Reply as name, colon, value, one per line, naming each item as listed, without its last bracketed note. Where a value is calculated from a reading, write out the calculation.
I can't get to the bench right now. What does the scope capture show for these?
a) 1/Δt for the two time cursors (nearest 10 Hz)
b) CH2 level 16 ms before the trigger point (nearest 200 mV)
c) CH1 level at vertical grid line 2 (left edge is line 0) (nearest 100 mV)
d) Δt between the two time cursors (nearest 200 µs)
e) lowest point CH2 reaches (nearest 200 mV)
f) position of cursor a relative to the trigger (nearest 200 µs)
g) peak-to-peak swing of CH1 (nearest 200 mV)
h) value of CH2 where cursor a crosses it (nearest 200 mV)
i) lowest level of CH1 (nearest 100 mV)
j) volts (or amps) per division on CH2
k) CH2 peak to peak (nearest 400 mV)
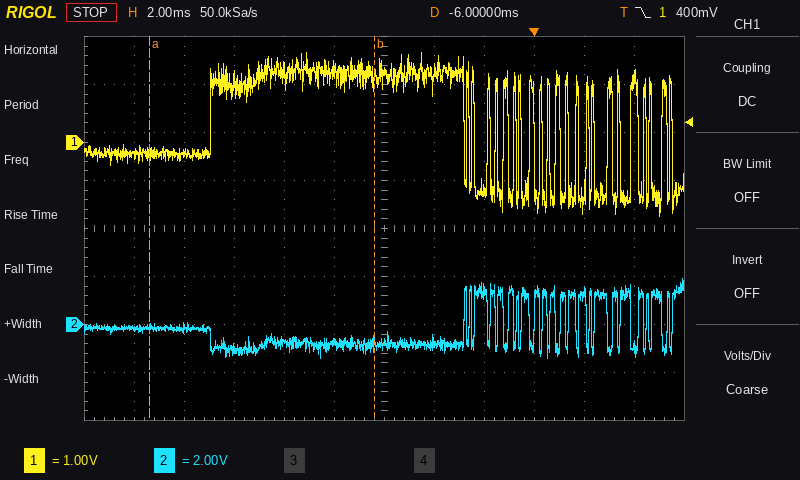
1/Δt for the two time cursors: 1 / 9.0 ms ≈ 110 Hz
CH2 level 16 ms before the trigger point: -200 mV
CH1 level at vertical grid line 2 (left edge is line 0): -200 mV
Δt between the two time cursors: 9.0 ms
lowest point CH2 reaches: -1.4 V
position of cursor a relative to the trigger: -15.4 ms
peak-to-peak swing of CH1: 3.4 V
value of CH2 where cursor a crosses it: 0.0 V
lowest level of CH1: -1.5 V
volts (or amps) per division on CH2: 2 V
CH2 peak to peak: 3.2 V
